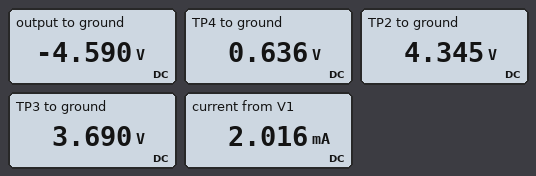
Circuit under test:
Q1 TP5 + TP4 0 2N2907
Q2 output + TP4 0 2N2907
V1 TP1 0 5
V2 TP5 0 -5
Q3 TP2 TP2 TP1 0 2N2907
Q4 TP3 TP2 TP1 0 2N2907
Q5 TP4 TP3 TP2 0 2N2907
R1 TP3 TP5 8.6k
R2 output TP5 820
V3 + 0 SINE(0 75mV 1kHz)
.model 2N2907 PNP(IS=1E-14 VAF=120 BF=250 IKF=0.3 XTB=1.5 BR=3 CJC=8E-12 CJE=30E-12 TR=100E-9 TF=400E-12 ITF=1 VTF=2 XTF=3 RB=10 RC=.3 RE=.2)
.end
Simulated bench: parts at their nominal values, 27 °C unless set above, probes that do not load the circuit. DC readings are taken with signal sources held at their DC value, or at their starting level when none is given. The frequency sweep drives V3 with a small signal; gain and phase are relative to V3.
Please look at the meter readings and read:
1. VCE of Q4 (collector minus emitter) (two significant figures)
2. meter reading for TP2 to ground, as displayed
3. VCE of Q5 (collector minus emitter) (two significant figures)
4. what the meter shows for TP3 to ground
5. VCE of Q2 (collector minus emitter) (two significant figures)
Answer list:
-1.3 V
4.345 V
-3.7 V
3.690 V
-5.2 V
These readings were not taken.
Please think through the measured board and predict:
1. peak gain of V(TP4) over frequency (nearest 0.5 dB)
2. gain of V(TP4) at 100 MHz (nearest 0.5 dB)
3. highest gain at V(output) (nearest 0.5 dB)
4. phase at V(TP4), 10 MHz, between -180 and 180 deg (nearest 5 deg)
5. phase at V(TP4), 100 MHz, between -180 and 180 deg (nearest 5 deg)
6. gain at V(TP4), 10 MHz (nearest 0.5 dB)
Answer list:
0 dB
-0.5 dB
0 dB
0 deg
0 deg
0 dB
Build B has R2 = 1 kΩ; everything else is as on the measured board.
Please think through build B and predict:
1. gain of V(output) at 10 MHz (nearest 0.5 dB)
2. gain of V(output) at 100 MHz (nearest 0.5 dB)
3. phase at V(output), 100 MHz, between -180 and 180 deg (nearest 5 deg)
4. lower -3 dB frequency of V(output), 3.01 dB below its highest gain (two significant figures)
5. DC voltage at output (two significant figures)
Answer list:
-24.5 dB
-0.5 dB
40 deg
50 MHz
-4.5 V
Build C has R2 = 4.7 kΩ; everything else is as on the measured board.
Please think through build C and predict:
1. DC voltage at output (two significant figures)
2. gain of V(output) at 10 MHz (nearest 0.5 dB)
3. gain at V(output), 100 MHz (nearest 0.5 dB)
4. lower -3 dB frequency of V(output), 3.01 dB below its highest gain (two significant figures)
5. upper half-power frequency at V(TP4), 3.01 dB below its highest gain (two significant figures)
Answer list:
-2.7 V
-15.5 dB
0 dB
40 MHz
3.5 GHz
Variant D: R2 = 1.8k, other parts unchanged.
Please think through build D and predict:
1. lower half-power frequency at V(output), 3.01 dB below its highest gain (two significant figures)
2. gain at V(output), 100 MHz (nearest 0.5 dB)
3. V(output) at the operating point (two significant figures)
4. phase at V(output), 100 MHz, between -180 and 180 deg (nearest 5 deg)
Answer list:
43 MHz
-0.5 dB
-4.1 V
30 deg
